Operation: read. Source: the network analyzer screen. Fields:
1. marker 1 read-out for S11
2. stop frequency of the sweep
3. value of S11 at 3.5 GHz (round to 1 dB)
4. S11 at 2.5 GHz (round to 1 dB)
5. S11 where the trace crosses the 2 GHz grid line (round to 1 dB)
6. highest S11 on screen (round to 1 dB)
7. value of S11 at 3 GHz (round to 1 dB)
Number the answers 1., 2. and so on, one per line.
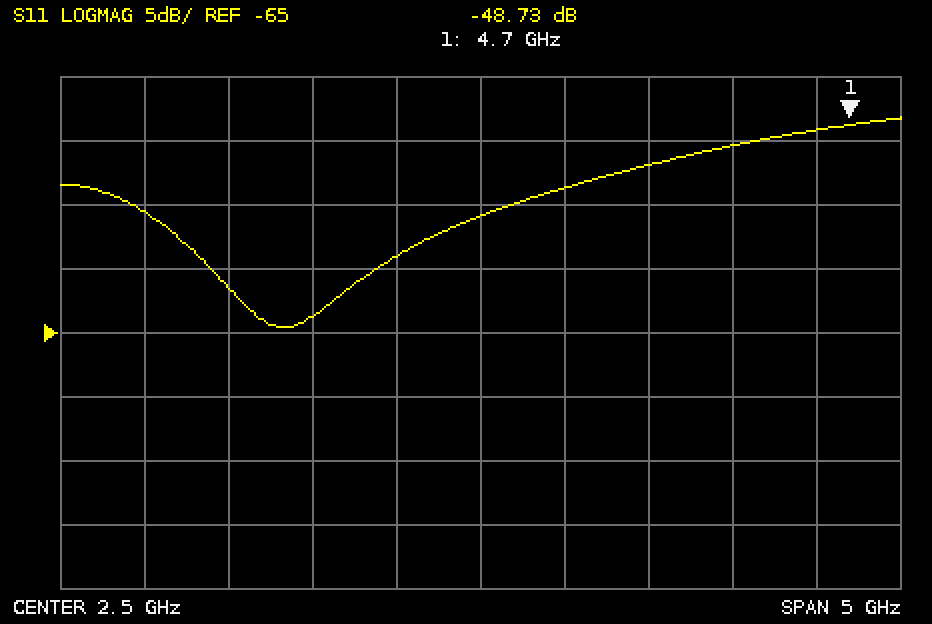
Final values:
1. -48.73 dB
2. 5 GHz
3. -52 dB
4. -56 dB
5. -59 dB
6. -48 dB
7. -54 dB
